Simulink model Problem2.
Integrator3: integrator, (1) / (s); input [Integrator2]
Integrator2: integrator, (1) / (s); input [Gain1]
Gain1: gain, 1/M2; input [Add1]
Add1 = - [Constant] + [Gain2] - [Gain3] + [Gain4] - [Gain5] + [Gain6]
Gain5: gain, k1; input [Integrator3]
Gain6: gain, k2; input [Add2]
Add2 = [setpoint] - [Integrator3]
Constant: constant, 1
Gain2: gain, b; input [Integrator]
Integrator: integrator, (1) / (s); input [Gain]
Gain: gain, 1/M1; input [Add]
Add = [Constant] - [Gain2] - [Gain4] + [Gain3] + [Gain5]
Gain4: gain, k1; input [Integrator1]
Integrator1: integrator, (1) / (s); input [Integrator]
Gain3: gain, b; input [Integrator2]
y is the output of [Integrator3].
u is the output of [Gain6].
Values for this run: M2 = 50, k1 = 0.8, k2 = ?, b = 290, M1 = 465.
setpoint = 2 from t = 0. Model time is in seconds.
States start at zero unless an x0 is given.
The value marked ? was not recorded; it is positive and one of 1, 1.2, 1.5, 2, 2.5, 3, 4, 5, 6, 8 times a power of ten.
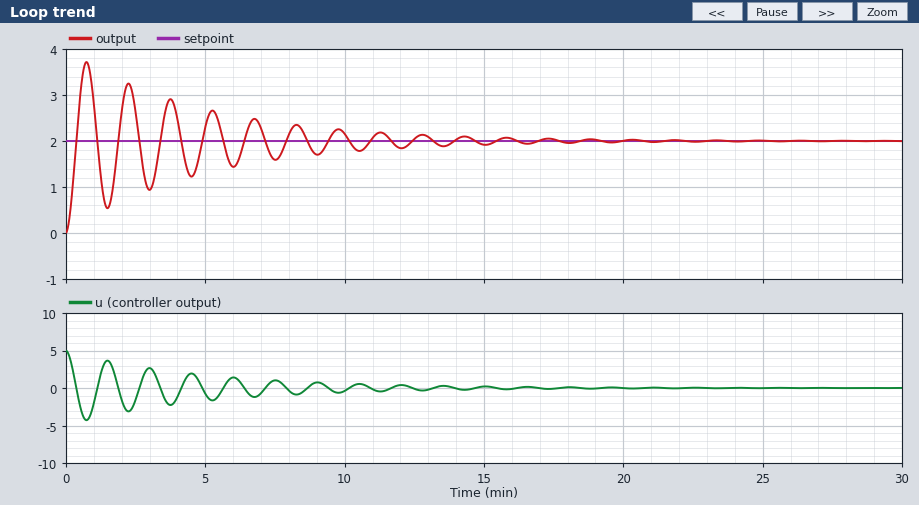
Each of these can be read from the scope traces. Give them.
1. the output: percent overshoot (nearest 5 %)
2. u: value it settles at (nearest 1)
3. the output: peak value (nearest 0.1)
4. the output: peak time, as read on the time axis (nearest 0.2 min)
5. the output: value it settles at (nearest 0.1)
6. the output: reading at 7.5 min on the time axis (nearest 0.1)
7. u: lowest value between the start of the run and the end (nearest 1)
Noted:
85 %
0
3.7
0.8 min
2.0
1.6
-4
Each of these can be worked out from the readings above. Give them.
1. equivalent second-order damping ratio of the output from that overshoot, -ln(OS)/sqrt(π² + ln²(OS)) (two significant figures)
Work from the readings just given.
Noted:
0.052
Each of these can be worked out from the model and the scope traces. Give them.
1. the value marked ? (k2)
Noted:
2.5
